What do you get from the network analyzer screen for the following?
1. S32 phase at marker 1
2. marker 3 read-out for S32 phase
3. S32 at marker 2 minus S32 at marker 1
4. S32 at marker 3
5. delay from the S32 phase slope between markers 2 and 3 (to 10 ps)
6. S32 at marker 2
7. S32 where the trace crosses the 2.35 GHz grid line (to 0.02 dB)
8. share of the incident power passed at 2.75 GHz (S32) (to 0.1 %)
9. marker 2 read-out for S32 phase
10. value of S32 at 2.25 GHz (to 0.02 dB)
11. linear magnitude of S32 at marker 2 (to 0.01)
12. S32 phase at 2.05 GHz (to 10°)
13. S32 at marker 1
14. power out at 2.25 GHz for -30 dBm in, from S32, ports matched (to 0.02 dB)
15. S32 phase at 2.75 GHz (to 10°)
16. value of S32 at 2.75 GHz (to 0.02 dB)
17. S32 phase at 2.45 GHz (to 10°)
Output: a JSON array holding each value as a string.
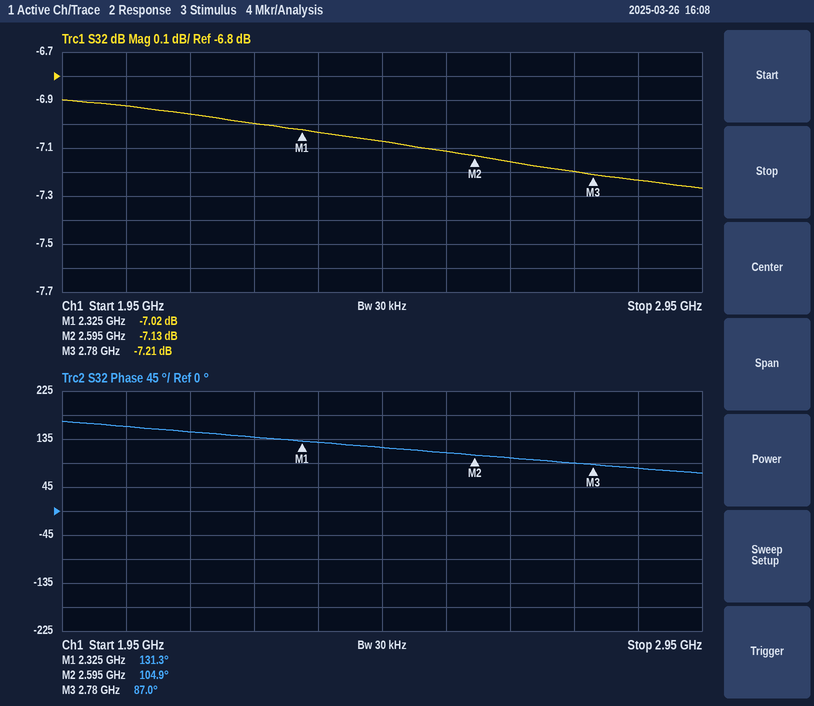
["131.3°", "87.0°", "-0.11 dB", "-7.21 dB", "270 ps", "-7.13 dB", "-7.04 dB", "19.1 %", "104.9°", "-7.00 dB", "0.44", "160°", "-7.02 dB", "-37.00 dBm", "90°", "-7.20 dB", "120°"]
